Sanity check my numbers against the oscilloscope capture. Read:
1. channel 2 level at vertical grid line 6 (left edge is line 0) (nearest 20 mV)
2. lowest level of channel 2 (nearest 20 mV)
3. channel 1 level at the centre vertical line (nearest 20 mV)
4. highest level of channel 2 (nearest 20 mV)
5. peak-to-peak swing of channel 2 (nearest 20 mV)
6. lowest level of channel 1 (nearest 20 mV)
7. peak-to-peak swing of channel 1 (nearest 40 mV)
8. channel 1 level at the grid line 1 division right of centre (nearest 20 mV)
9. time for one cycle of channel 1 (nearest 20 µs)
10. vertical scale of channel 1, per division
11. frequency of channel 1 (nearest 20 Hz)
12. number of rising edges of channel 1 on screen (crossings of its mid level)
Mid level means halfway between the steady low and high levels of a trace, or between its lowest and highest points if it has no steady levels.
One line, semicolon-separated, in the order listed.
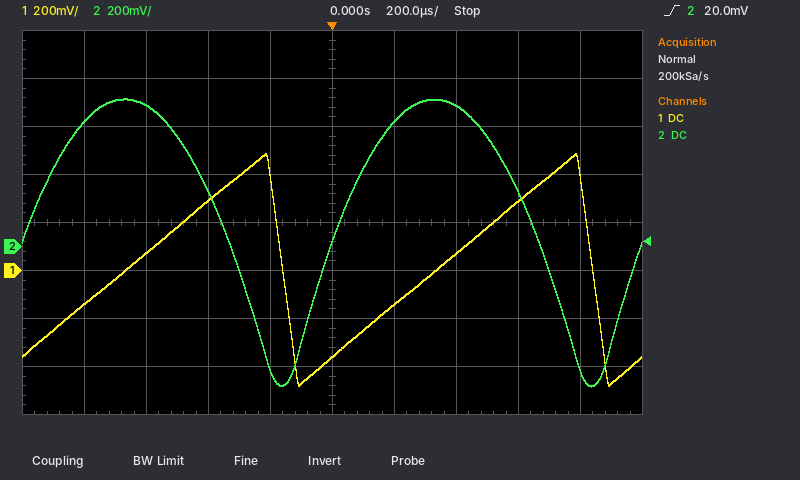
520 mV; -580 mV; -360 mV; 620 mV; 1.20 V; -480 mV; 960 mV; -140 mV; 1.00 ms; 200 mV; 1.00 kHz; 2
